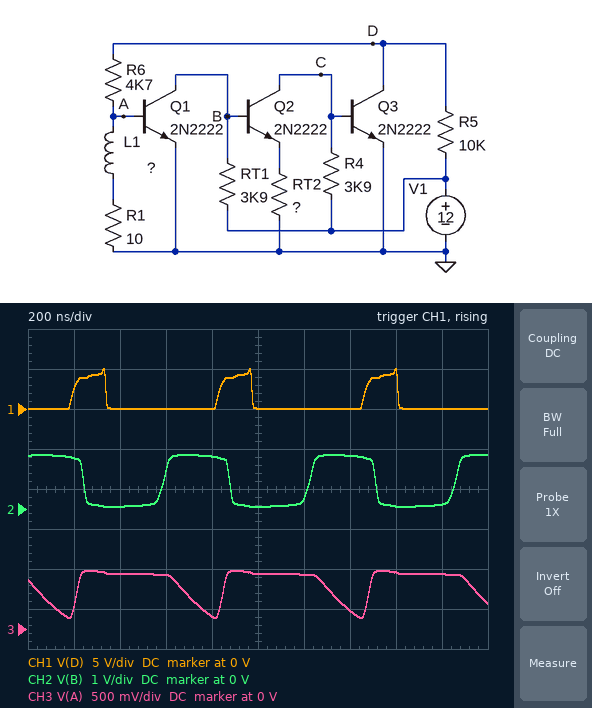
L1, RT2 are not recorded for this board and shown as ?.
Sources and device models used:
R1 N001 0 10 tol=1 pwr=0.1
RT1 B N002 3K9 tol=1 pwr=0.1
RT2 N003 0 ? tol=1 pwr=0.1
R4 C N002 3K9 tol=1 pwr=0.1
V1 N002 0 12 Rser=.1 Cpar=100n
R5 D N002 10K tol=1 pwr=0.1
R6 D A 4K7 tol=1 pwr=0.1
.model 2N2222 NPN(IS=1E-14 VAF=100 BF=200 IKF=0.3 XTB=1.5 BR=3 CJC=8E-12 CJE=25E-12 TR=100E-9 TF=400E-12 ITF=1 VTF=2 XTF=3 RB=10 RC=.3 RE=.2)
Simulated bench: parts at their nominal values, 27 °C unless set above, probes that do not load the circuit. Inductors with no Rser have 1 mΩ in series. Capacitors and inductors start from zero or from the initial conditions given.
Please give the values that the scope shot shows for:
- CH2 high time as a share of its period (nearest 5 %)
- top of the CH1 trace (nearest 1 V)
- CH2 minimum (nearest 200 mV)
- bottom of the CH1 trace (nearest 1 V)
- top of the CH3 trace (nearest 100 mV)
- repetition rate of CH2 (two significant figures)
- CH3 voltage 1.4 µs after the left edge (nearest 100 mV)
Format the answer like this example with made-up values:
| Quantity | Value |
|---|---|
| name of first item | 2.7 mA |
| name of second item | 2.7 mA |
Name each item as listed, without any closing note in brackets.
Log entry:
| Quantity | Value |
|---|---|
| CH2 high time as a share of its period | 45 % |
| top of the CH1 trace | 5 V |
| CH2 minimum | 0 V |
| bottom of the CH1 trace | 0 V |
| top of the CH3 trace | 700 mV |
| repetition rate of CH2 | 1.6 MHz |
| CH3 voltage 1.4 µs after the left edge | 200 mV |
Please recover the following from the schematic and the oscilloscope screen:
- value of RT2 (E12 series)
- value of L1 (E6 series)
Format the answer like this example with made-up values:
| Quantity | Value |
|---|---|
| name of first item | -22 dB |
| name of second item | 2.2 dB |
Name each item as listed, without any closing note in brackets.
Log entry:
| Quantity | Value |
|---|---|
| value of RT2 | 82 Ω |
| value of L1 | 680 mH |
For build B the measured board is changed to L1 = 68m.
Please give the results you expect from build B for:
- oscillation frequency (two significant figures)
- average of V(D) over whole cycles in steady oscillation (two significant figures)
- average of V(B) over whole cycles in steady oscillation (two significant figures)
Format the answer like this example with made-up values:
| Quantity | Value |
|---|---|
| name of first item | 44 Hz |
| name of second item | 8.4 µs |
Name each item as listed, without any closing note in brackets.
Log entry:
| Quantity | Value |
|---|---|
| oscillation frequency | 2.1 MHz |
| average of V(D) over whole cycles in steady oscillation | 1.6 V |
| average of V(B) over whole cycles in steady oscillation | 770 mV |
